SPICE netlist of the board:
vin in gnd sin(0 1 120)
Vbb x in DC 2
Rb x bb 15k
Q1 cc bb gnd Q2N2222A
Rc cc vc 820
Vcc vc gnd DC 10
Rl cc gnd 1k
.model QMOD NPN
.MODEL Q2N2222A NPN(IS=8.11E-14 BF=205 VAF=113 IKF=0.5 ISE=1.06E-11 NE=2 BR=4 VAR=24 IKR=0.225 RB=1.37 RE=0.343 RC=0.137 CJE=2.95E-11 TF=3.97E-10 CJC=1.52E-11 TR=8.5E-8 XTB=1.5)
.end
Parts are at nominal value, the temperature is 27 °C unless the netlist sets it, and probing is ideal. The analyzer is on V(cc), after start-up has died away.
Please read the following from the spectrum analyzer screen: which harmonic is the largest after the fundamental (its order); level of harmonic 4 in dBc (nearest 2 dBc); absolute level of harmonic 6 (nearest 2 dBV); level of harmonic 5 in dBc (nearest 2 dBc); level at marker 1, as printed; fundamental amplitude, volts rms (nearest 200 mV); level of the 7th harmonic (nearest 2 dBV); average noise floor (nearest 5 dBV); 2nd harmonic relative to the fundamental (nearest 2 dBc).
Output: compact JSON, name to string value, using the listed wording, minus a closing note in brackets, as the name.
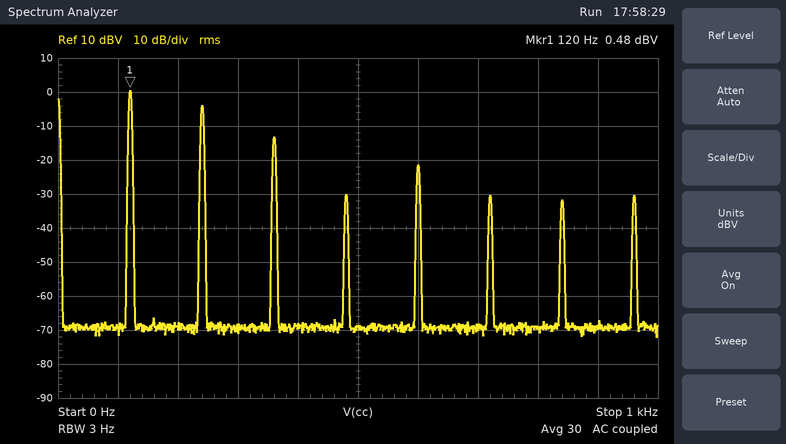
{"which harmonic is the largest after the fundamental": "2", "level of harmonic 4 in dBc": "-30 dBc", "absolute level of harmonic 6": "-30 dBV", "level of harmonic 5 in dBc": "-22 dBc", "level at marker 1, as printed": "0.48 dBV", "fundamental amplitude, volts rms": "1.0 V", "level of the 7th harmonic": "-32 dBV", "average noise floor": "-70 dBV", "2nd harmonic relative to the fundamental": "-4 dBc"}
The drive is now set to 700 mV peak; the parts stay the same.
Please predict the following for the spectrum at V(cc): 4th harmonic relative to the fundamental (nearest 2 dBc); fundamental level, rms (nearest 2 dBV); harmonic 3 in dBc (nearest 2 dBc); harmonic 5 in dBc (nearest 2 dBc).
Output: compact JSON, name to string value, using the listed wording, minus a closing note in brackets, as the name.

{"4th harmonic relative to the fundamental": "-24 dBc", "fundamental level, rms": "-6 dBV", "harmonic 3 in dBc": "-10 dBc", "harmonic 5 in dBc": "-24 dBc"}
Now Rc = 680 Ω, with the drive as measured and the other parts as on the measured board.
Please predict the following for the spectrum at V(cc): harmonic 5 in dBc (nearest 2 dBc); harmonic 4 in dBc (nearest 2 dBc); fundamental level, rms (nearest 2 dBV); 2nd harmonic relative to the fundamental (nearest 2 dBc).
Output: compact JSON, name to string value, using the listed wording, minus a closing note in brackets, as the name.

{"harmonic 5 in dBc": "-28 dBc", "harmonic 4 in dBc": "-22 dBc", "fundamental level, rms": "2 dBV", "2nd harmonic relative to the fundamental": "-6 dBc"}
